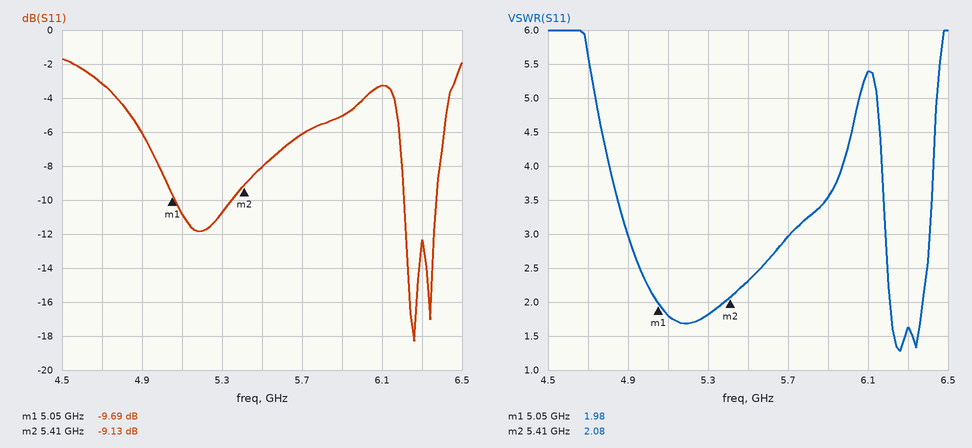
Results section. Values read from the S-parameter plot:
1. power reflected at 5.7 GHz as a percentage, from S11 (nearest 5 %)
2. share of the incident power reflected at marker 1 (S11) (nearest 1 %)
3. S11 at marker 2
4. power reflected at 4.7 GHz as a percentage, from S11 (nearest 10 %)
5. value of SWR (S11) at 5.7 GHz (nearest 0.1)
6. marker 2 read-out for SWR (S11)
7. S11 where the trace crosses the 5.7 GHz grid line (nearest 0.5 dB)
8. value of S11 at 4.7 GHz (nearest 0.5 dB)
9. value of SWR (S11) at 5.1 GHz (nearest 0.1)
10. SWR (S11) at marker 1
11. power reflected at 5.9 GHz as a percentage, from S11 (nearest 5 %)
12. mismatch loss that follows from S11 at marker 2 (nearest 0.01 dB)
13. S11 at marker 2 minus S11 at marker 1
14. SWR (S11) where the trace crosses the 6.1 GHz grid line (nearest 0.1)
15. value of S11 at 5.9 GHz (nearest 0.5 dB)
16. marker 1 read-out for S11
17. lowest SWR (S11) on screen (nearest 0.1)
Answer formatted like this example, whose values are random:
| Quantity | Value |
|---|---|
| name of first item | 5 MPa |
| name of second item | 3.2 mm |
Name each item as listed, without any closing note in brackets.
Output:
| Quantity | Value |
|---|---|
| power reflected at 5.7 GHz as a percentage, from S11 | 25 % |
| share of the incident power reflected at marker 1 (S11) | 11 % |
| S11 at marker 2 | -9.13 dB |
| power reflected at 4.7 GHz as a percentage, from S11 | 50 % |
| value of SWR (S11) at 5.7 GHz | 3.0 |
| marker 2 read-out for SWR | 2.08 |
| S11 where the trace crosses the 5.7 GHz grid line | -6.0 dB |
| value of S11 at 4.7 GHz | -3.0 dB |
| value of SWR (S11) at 5.1 GHz | 1.8 |
| SWR (S11) at marker 1 | 1.98 |
| power reflected at 5.9 GHz as a percentage, from S11 | 30 % |
| mismatch loss that follows from S11 at marker 2 | 0.57 dB |
| S11 at marker 2 minus S11 at marker 1 | 0.56 dB |
| SWR (S11) where the trace crosses the 6.1 GHz grid line | 5.4 |
| value of S11 at 5.9 GHz | -5.0 dB |
| marker 1 read-out for S11 | -9.69 dB |
| lowest SWR (S11) on screen | 1.3 |
